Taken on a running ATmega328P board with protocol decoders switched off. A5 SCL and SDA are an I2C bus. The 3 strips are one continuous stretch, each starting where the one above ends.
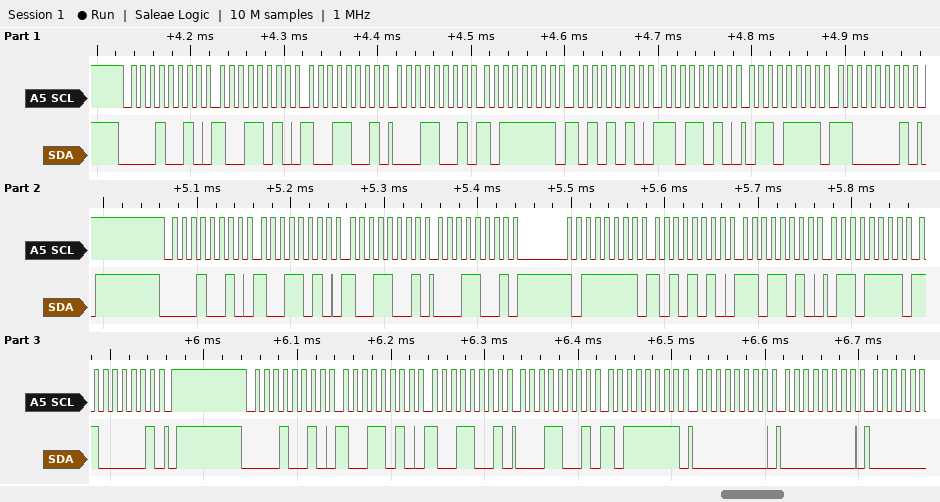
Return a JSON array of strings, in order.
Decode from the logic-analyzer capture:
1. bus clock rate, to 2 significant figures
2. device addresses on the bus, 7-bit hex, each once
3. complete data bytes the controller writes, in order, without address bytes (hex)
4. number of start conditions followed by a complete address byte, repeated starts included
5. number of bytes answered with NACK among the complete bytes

["100 kHz", "0x09", "9A 99 19 BF AA DA 6F C1 9A 99 19 BF AA DA 6F C1 9A 99 19 BF 00 00", "3", "0"]
